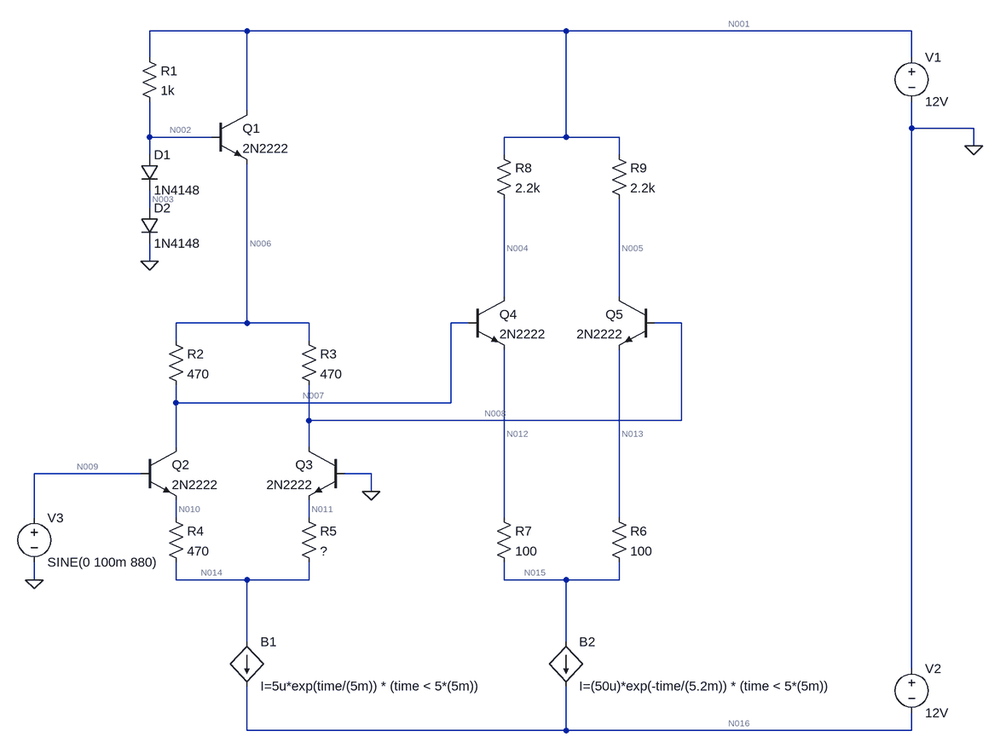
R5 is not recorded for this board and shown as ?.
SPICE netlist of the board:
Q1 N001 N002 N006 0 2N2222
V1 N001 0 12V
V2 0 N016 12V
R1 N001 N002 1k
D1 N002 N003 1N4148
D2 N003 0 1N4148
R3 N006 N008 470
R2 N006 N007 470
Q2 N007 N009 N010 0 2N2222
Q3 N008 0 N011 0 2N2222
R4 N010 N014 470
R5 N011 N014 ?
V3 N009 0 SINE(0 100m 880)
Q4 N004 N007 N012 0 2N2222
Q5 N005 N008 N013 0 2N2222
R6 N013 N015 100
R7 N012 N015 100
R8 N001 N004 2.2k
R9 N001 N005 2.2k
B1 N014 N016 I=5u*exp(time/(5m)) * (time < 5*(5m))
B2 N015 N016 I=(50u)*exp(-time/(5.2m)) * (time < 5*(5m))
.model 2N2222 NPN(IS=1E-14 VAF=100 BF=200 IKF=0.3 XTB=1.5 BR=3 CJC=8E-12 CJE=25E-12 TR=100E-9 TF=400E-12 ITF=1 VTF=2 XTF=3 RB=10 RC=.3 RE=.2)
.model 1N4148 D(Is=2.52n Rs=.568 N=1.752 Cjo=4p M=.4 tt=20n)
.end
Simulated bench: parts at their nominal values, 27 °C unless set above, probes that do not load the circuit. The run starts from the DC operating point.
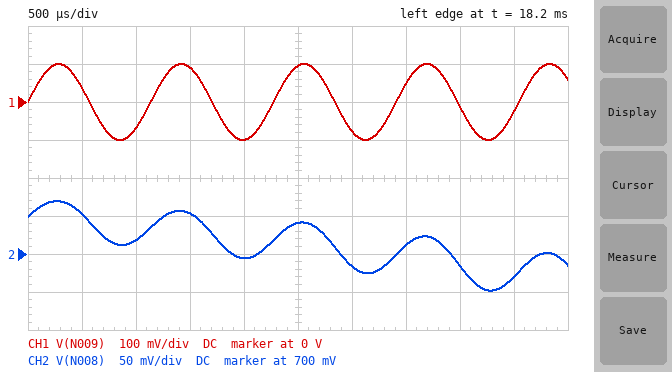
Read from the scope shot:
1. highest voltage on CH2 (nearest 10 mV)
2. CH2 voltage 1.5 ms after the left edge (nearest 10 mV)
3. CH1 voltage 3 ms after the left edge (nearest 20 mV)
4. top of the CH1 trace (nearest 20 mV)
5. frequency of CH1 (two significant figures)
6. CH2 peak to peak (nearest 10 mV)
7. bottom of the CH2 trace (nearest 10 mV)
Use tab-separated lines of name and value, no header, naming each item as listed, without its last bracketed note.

highest voltage on CH2	770 mV
CH2 voltage 1.5 ms after the left edge	750 mV
CH1 voltage 3 ms after the left edge	-80 mV
top of the CH1 trace	100 mV
frequency of CH1	880 Hz
CH2 peak to peak	120 mV
bottom of the CH2 trace	650 mV
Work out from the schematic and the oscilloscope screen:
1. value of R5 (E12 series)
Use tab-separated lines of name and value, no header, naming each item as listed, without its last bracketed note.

value of R5	820 Ω
